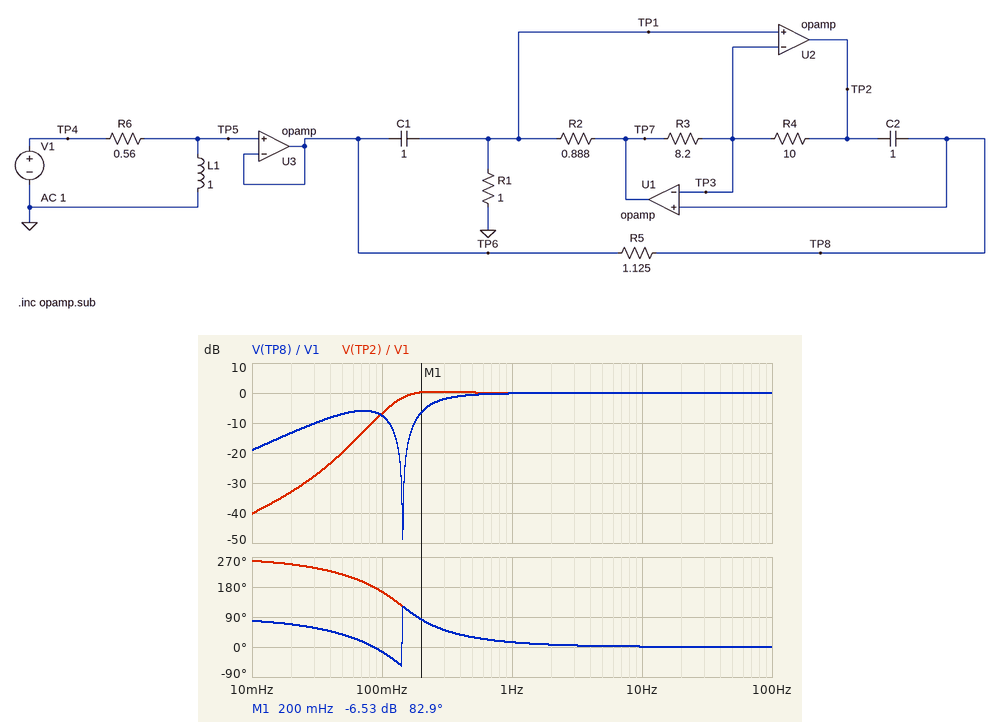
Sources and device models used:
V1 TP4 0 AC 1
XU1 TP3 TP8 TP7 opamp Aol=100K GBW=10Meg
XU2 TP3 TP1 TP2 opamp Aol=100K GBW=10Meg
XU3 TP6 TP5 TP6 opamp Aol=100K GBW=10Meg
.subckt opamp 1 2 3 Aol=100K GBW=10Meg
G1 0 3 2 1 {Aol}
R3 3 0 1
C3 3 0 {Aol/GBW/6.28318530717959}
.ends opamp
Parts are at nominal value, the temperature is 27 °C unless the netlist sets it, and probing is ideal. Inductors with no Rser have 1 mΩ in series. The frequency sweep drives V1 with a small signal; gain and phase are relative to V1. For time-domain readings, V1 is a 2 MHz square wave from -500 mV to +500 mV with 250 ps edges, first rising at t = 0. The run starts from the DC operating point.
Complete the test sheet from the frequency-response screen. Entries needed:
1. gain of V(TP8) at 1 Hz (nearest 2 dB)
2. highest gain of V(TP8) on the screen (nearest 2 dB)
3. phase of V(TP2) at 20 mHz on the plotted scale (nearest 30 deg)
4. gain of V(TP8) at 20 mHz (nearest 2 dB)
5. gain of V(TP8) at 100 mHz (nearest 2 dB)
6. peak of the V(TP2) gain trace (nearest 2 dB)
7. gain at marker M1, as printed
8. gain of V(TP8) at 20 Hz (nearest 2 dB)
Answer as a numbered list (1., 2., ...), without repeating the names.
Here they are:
1. 0 dB
2. 0 dB
3. 240 deg
4. -14 dB
5. -8 dB
6. 0 dB
7. -6.53 dB
8. 0 dB
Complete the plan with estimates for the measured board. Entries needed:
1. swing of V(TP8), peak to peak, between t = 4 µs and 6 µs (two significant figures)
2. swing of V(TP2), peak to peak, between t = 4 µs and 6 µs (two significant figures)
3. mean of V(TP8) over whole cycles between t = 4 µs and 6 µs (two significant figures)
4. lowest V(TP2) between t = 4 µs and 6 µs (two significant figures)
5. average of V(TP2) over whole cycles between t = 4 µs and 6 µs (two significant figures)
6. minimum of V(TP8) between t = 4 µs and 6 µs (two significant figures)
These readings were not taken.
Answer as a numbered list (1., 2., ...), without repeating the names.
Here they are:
1. 1.3 V
2. 1.3 V
3. 500 mV
4. -150 mV
5. 500 mV
6. -150 mV
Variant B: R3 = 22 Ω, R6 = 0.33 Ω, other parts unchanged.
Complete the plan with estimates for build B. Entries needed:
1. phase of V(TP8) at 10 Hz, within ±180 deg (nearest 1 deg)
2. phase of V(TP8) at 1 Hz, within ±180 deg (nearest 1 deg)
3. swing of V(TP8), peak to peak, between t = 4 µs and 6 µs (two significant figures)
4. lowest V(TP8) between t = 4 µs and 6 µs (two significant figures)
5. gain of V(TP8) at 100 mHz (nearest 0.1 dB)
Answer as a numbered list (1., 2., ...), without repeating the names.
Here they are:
1. 1 deg
2. 13 deg
3. 1.2 V
4. -120 mV
5. -1.6 dB
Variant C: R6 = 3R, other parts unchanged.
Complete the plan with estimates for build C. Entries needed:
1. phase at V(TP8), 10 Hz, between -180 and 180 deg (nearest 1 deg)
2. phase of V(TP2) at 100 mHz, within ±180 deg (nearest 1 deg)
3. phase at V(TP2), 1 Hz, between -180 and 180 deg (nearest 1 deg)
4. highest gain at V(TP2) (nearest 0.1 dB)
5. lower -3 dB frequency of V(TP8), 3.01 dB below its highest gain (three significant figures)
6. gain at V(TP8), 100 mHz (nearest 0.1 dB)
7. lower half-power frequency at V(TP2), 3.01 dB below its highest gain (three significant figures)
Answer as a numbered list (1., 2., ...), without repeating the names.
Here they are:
1. 4 deg
2. -158 deg
3. 35 deg
4. 0 dB
5. 531 mHz
6. -18.8 dB
7. 436 mHz
